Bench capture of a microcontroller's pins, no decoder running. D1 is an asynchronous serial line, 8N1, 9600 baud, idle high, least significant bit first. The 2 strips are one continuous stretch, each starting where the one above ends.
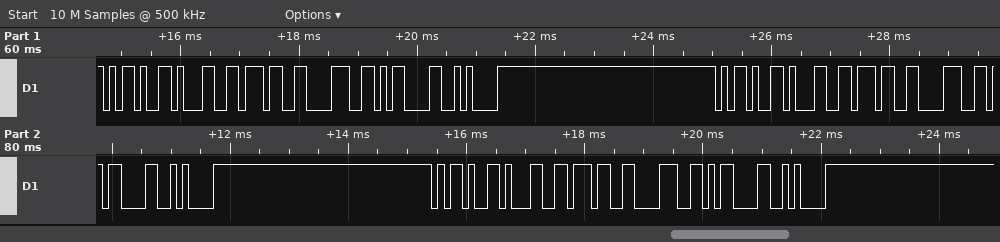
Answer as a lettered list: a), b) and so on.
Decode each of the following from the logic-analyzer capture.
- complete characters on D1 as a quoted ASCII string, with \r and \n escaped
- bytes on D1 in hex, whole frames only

a) "-178\r\n-178\r\n-178\r\n"
b) 2D 31 37 38 0D 0A 2D 31 37 38 0D 0A 2D 31 37 38 0D 0A
